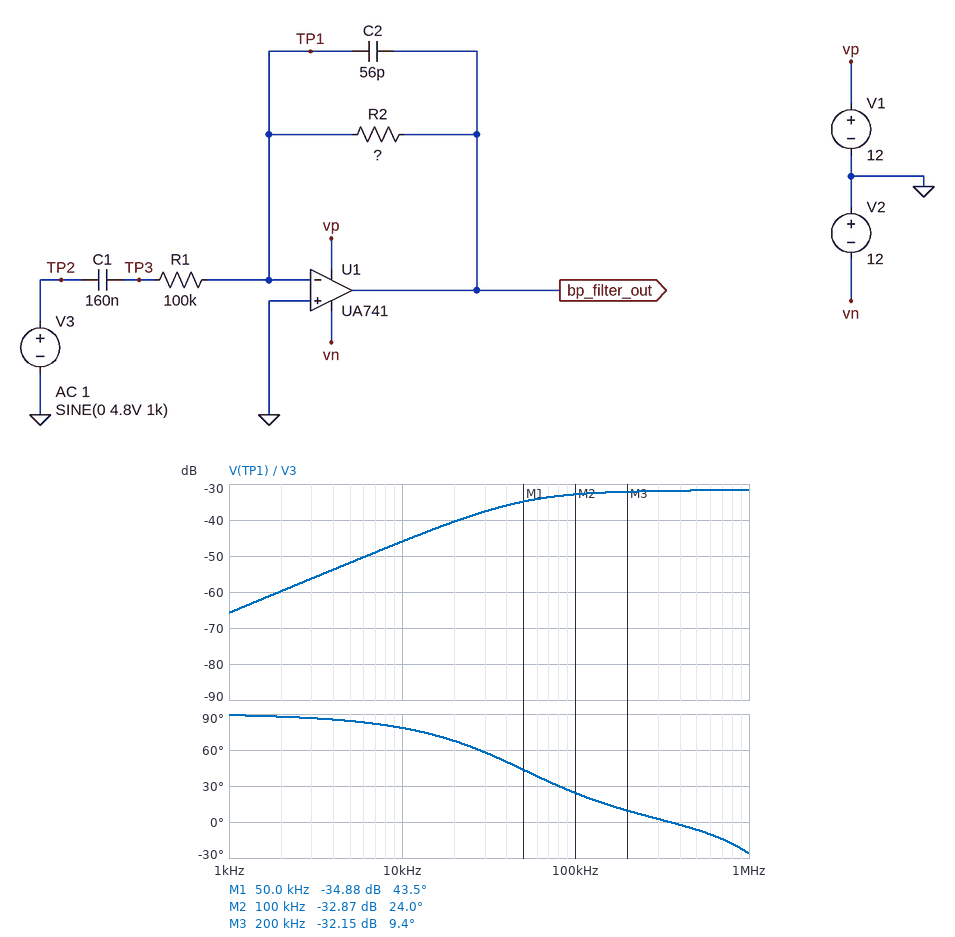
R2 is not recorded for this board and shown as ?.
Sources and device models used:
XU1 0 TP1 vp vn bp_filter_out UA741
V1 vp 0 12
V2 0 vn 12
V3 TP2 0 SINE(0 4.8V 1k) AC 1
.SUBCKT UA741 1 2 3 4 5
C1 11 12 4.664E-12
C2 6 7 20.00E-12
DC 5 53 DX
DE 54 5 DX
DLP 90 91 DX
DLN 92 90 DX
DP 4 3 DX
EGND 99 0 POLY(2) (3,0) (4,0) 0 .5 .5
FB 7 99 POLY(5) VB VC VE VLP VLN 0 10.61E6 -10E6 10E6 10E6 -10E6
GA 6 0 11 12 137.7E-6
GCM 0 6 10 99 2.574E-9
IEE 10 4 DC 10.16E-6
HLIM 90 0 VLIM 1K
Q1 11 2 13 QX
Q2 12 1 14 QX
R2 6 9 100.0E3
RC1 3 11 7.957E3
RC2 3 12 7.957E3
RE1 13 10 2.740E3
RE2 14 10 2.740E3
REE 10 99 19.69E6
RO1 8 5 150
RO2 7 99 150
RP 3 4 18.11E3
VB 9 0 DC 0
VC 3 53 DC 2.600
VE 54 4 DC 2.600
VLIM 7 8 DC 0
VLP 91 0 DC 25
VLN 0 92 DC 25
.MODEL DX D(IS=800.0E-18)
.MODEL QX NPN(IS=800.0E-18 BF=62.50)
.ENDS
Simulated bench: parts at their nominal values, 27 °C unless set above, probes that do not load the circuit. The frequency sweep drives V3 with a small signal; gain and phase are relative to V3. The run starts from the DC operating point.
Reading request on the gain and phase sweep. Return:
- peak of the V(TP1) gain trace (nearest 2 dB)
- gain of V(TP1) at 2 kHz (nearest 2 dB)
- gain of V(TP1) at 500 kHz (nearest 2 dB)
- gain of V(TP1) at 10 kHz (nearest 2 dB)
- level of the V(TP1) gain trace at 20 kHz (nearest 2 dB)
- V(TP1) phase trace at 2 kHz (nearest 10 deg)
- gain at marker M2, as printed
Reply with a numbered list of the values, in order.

1. -32 dB
2. -60 dB
3. -32 dB
4. -46 dB
5. -40 dB
6. 90 deg
7. -32.87 dB
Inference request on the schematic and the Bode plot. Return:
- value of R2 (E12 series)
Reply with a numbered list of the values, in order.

1. 56 kΩ
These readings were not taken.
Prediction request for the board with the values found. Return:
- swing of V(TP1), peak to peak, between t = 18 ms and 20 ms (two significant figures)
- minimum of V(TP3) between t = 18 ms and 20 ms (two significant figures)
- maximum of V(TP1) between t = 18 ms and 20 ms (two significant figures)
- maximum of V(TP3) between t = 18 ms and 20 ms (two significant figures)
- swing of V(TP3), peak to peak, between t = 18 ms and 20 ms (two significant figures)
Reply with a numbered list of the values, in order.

1. 4.9 mV
2. -4.8 V
3. 2.5 mV
4. 4.8 V
5. 9.6 V
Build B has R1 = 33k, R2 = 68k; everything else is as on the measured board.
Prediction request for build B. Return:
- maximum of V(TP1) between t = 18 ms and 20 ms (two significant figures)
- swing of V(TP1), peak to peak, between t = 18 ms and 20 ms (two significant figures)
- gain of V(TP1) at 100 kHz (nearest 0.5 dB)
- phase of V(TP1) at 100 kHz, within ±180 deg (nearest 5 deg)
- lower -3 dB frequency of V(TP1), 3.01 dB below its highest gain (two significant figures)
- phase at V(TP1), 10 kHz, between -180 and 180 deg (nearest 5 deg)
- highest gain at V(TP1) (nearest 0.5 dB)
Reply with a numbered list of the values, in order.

1. 9.1 mV
2. 18 mV
3. -23.5 dB
4. 20 deg
5. 42 kHz
6. 75 deg
7. -22.5 dB
